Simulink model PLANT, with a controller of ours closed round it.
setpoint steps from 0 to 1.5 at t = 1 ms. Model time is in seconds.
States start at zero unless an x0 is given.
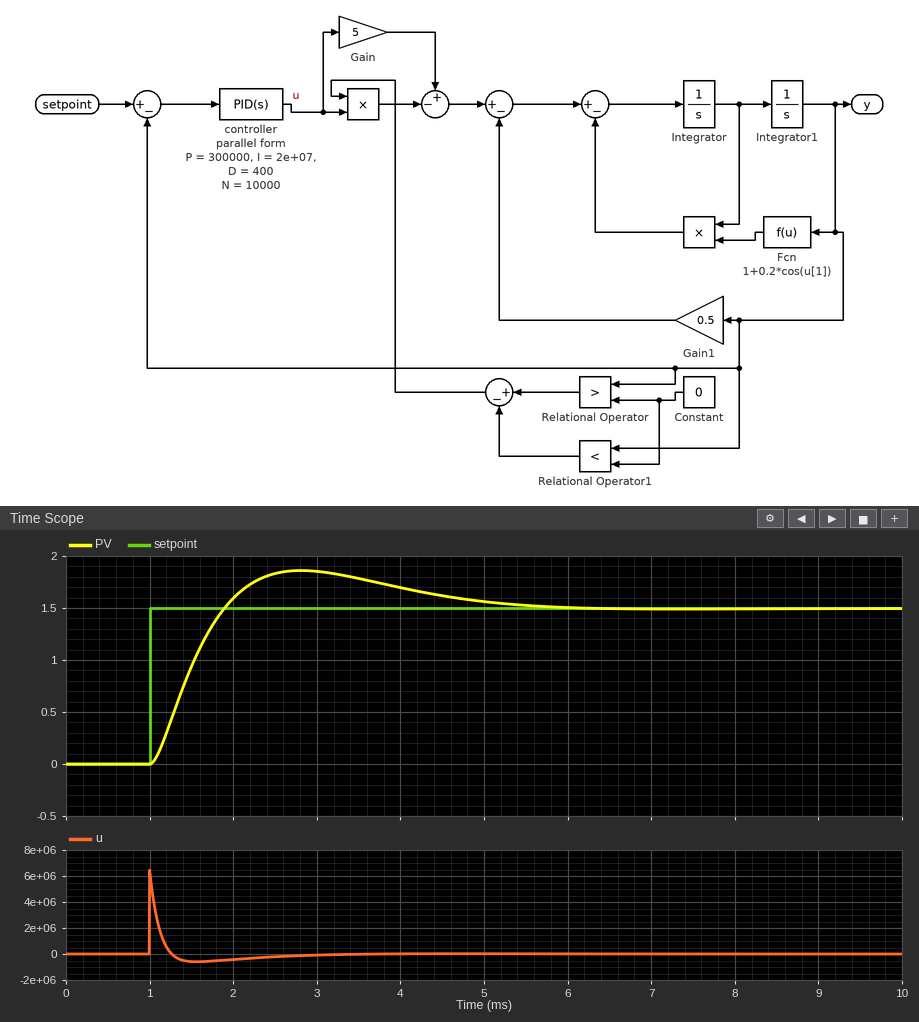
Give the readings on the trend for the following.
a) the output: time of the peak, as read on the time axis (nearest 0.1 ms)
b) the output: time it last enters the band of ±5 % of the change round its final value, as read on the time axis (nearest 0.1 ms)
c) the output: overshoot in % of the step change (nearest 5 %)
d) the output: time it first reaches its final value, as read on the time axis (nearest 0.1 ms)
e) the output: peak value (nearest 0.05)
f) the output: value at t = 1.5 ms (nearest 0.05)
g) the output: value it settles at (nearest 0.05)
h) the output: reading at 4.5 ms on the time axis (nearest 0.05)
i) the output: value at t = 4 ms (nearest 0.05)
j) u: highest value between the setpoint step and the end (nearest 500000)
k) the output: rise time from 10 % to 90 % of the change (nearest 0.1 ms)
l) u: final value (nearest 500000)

2.8 ms
4.9 ms
25 %
1.9 ms
1.85
0.95
1.50
1.60
1.70
6500000
0.6 ms
0
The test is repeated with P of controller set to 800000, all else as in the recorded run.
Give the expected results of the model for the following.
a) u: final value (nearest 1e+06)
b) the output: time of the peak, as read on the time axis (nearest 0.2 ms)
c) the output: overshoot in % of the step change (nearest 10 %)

0
2.2 ms
40 %
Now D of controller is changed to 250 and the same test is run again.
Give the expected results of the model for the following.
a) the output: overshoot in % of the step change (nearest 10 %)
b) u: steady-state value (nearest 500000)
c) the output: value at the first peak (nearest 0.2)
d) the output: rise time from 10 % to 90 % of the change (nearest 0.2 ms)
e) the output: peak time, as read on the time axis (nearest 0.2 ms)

40 %
0
2.0
0.8 ms
3.2 ms
